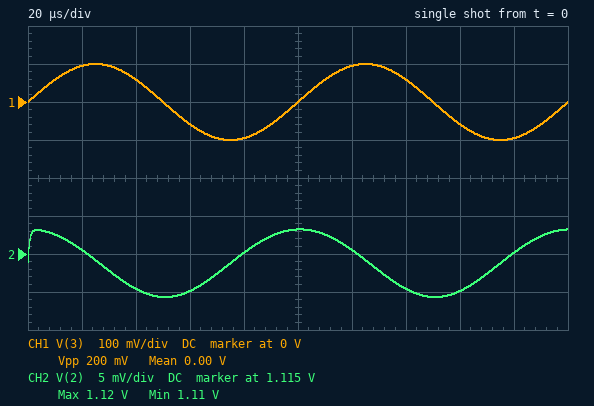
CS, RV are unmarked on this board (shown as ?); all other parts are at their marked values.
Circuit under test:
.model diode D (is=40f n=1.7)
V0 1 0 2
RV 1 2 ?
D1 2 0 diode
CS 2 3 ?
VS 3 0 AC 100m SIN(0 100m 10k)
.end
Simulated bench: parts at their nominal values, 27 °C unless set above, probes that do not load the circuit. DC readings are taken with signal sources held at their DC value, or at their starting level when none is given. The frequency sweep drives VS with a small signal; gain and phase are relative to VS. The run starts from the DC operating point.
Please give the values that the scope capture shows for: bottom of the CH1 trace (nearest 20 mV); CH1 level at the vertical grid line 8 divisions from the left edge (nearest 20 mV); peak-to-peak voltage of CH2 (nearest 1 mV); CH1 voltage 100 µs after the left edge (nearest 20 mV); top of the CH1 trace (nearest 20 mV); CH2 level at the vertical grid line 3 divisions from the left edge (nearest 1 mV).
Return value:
-100 mV
-60 mV
9 mV
0 V
100 mV
1.110 V
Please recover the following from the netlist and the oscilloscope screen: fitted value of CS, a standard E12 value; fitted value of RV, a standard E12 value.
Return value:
68 nF
220 Ω
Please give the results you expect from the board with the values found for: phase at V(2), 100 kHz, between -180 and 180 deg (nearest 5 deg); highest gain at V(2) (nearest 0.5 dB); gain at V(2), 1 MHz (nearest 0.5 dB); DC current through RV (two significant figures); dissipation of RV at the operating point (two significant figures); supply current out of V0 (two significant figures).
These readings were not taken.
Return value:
65 deg
0 dB
0 dB
4.0 mA
3.6 mW
4.0 mA
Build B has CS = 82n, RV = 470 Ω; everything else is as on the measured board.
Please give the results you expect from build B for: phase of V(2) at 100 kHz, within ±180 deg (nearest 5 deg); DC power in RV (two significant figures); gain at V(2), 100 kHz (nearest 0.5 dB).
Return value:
40 deg
1.8 mW
-2.5 dB
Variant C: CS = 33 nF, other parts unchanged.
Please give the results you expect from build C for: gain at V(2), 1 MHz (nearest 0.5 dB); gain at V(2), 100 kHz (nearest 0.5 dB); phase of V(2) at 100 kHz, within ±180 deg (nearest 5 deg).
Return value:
-1.0 dB
-13.5 dB
80 deg
